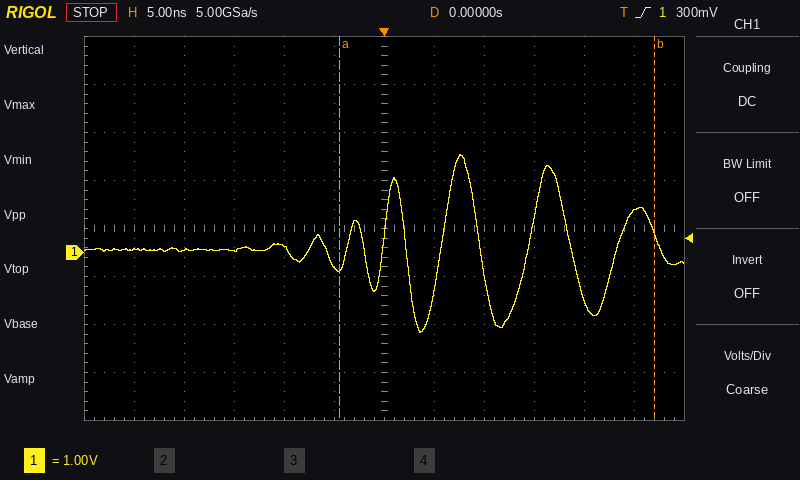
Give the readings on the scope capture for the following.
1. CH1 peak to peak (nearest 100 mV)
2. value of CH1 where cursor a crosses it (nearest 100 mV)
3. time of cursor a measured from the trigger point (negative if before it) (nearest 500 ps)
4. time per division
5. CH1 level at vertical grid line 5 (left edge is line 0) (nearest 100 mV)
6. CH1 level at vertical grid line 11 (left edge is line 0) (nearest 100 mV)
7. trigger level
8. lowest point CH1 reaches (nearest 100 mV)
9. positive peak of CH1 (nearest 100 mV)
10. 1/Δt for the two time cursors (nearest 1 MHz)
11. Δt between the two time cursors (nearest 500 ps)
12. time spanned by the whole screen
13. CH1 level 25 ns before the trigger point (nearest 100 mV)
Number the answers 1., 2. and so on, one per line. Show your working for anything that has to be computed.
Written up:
1. 2.0 V − (-1.7 V) = 3.7 V
2. -300 mV
3. -4.5 ns
4. 5 ns
5. -300 mV
6. 900 mV
7. 300 mV
8. -1.7 V
9. 2.0 V
10. 1 / 31.5 ns ≈ 32 MHz
11. 31.5 ns
12. 60 ns
13. 100 mV
